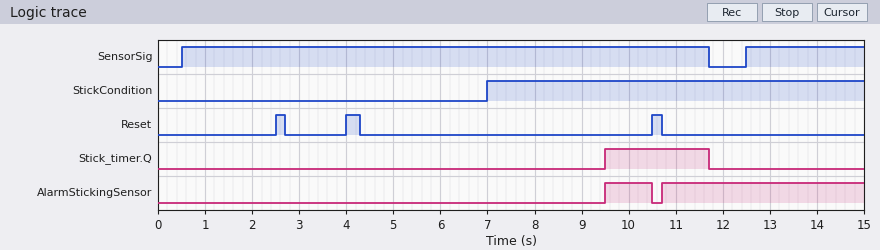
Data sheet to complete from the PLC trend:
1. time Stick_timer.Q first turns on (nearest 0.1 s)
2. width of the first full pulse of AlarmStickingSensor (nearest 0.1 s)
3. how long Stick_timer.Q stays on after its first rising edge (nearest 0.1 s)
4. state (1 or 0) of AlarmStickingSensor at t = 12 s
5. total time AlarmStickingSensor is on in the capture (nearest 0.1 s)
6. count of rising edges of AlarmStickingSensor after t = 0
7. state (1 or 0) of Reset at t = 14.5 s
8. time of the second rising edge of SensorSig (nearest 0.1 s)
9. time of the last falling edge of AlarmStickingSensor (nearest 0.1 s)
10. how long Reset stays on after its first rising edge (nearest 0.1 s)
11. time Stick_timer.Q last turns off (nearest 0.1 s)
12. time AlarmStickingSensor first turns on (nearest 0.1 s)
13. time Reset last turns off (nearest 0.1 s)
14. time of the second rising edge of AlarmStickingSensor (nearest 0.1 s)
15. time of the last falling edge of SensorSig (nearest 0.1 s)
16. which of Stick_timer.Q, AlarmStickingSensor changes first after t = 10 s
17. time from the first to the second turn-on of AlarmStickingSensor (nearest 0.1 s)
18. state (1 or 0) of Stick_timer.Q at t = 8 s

9.5 s
1.0 s
2.2 s
1
5.3 s
2
0
12.5 s
10.5 s
0.2 s
11.7 s
9.5 s
10.7 s
10.7 s
11.7 s
AlarmStickingSensor
1.2 s
0
